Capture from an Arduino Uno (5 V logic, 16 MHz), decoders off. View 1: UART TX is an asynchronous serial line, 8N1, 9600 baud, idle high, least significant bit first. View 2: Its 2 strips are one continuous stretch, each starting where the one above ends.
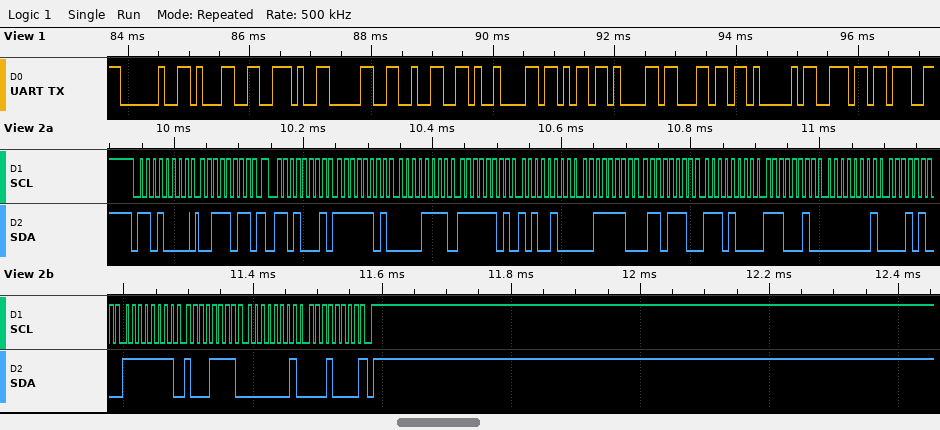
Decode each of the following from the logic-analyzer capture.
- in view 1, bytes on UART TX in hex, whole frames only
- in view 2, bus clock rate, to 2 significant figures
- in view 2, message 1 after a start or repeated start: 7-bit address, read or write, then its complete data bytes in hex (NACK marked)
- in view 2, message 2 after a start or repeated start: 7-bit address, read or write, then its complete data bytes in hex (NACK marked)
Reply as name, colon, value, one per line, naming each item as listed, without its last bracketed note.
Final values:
in view 1, bytes on UART TX in hex, whole frames only: 0x20 0x31 0x2E 0x30 0x32 0x09 0x6B 0x61 0x6C 0x41 0x6E
in view 2, bus clock rate, to 2 significant figures: 100 kHz
in view 2, message 1 after a start or repeated start: 7-bit address, read or write, then its complete data bytes in hex: 0x68 write: 3B
in view 2, message 2 after a start or repeated start: 7-bit address, read or write, then its complete data bytes in hex: 0x68 read: FD 0F FD A4 3E 6E E8 E2 01 14 FF 8F 01 10 NACK
